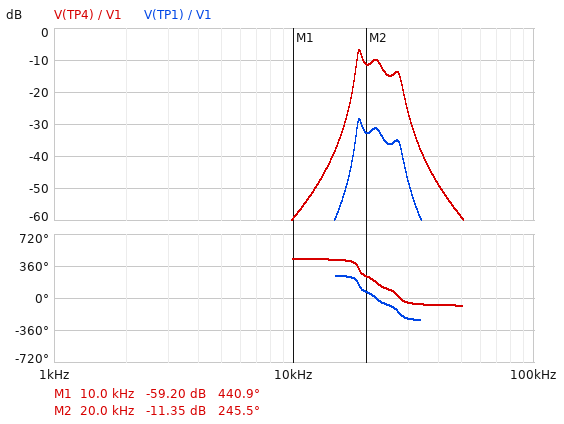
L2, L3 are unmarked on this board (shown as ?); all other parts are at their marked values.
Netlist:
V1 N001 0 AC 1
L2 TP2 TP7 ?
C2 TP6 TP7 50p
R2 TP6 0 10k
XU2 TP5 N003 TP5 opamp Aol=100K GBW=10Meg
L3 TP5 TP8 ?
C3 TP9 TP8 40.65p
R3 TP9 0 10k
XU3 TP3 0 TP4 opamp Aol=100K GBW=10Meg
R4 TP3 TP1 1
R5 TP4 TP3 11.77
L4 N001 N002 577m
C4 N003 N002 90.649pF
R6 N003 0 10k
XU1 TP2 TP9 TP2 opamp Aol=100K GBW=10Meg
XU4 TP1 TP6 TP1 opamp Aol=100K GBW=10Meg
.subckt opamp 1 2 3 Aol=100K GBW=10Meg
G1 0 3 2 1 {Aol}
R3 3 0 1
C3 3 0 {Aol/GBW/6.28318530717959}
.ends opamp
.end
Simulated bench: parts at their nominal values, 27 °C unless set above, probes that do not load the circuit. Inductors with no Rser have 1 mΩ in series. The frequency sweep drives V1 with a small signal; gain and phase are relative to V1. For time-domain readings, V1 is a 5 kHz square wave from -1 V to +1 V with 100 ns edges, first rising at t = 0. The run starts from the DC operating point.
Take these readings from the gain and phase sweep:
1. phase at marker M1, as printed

440.9 deg
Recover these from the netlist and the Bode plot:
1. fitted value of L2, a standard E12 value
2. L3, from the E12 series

680 mH
1.8 H
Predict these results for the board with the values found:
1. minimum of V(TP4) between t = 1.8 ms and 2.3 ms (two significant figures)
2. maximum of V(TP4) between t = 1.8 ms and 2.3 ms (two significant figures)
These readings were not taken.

-49 mV
49 mV
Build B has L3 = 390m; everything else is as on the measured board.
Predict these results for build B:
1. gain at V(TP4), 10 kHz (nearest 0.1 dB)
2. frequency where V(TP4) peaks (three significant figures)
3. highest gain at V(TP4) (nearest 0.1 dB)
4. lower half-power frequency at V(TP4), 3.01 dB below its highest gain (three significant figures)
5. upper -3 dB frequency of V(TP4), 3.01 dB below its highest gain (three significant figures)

-61.6 dB
27.2 kHz
-7.5 dB
25.9 kHz
28.4 kHz
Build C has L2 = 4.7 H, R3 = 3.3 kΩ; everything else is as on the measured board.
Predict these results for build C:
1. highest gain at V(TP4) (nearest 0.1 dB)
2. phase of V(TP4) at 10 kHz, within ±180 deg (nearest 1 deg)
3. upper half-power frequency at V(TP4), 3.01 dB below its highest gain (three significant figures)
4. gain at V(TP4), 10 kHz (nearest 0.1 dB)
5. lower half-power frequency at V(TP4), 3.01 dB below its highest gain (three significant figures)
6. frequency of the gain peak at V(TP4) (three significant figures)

-19.3 dB
61 deg
18.8 kHz
-48.0 dB
18.5 kHz
18.6 kHz
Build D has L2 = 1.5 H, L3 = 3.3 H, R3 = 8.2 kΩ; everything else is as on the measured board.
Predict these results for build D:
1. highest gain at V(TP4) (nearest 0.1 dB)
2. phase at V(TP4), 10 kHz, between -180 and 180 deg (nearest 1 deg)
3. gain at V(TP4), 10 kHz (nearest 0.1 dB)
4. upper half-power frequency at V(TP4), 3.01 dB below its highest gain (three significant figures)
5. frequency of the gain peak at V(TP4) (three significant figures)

-14.5 dB
80 deg
-55.5 dB
19.0 kHz
18.4 kHz
